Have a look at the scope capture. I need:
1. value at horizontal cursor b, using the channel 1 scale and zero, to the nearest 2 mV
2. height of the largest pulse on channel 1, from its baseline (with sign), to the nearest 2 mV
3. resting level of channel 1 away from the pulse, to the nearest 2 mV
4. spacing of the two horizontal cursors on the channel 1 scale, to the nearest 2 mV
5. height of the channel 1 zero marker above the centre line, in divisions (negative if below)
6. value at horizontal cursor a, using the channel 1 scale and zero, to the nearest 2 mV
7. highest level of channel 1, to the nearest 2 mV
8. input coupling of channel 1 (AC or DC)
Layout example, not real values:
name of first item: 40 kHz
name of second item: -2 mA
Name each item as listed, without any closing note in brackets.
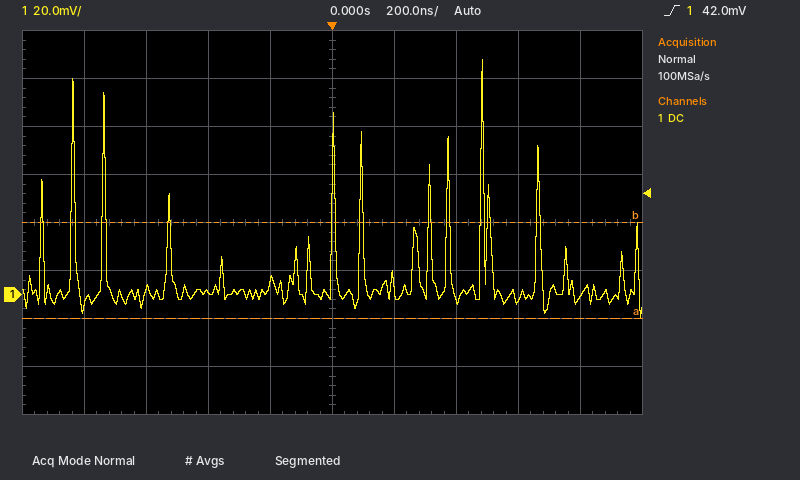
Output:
value at horizontal cursor b, using the channel 1 scale and zero, to the nearest 2 mV: 30 mV
height of the largest pulse on channel 1, from its baseline (with sign), to the nearest 2 mV: +98 mV
resting level of channel 1 away from the pulse, to the nearest 2 mV: 0 mV
spacing of the two horizontal cursors on the channel 1 scale, to the nearest 2 mV: 40 mV
height of the channel 1 zero marker above the centre line, in divisions: -1.5 div
value at horizontal cursor a, using the channel 1 scale and zero, to the nearest 2 mV: -10 mV
highest level of channel 1, to the nearest 2 mV: 98 mV
input coupling of channel 1: DC
